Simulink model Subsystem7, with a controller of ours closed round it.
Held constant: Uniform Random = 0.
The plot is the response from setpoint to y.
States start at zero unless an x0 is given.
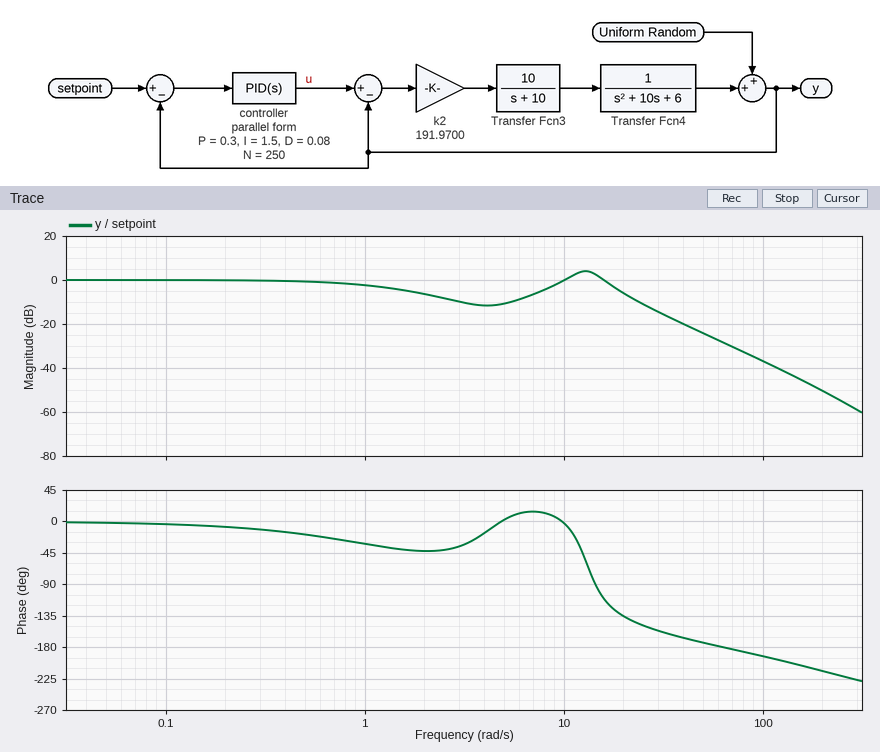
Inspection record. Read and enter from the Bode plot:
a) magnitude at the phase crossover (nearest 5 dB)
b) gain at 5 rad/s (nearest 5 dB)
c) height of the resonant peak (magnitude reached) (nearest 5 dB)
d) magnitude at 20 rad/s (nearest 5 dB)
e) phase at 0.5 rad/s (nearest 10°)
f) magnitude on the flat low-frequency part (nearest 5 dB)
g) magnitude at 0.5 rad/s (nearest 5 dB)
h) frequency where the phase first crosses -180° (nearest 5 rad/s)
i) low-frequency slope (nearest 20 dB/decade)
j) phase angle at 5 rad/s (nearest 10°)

-30 dB
-10 dB
5 dB
-5 dB
-20°
0 dB
0 dB
65 rad/s
0 dB/decade
0°
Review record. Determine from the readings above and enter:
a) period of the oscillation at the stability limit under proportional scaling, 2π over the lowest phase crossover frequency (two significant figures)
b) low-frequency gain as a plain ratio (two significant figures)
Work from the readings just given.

0.097 s
1.0
